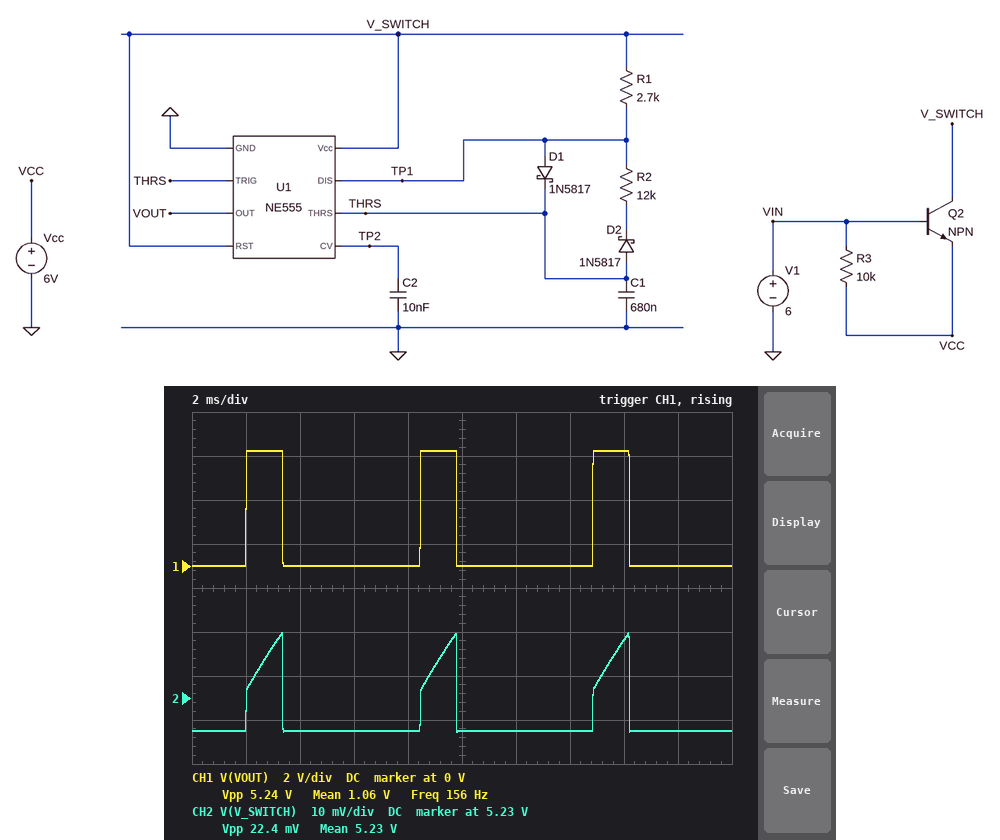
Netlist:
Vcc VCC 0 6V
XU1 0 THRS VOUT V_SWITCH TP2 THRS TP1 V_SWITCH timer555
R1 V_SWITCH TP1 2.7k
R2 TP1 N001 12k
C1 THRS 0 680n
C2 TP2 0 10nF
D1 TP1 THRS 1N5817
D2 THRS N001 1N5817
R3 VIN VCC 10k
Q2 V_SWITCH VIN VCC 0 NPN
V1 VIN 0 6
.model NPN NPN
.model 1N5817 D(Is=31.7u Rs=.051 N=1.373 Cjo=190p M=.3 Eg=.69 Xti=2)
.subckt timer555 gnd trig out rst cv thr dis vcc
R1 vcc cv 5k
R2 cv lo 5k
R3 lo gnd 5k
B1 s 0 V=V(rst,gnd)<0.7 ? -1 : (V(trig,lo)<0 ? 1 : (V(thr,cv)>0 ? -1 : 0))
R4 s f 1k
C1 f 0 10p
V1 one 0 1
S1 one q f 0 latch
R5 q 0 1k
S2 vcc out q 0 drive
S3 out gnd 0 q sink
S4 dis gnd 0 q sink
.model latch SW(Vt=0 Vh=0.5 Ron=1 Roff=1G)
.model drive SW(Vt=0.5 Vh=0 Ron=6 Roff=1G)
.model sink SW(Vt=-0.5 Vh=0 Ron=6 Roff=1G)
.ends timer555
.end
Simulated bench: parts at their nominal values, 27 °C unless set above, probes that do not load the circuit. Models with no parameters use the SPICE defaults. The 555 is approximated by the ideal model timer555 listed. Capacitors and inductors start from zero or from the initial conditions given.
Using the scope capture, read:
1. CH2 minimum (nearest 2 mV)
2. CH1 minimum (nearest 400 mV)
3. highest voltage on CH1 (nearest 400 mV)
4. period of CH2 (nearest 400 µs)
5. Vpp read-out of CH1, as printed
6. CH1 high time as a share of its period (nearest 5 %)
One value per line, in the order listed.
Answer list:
5.222 V
0 V
5.2 V
6.4 ms
5.24 V
20 %
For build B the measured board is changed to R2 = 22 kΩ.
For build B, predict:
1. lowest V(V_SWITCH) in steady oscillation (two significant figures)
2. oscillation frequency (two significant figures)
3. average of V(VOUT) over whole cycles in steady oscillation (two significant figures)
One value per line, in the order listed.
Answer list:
5.2 V
100 Hz
730 mV
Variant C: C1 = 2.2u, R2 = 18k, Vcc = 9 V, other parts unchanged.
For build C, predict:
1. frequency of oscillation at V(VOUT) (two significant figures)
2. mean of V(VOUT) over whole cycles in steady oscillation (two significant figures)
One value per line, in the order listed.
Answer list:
37 Hz
830 mV
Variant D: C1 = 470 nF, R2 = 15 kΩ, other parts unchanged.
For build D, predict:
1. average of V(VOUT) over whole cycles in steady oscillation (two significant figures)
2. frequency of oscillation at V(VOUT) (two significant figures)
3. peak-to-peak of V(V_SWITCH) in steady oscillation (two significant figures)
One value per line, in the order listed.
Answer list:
950 mV
190 Hz
22 mV
